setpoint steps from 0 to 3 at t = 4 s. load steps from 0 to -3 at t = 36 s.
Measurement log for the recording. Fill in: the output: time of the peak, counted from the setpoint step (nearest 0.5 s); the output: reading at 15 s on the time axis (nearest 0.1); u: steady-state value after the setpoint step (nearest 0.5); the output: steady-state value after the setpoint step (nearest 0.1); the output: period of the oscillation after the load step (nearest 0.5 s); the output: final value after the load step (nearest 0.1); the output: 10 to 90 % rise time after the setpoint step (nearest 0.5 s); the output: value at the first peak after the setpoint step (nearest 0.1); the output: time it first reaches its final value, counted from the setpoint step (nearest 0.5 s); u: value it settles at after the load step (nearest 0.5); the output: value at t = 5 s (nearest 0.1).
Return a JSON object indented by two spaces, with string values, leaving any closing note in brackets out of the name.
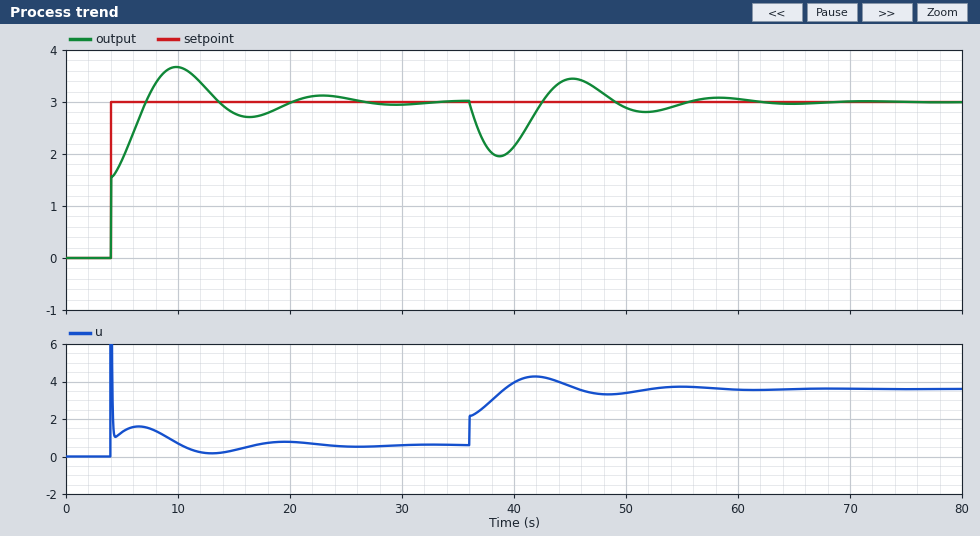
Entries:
{
  "the output: time of the peak, counted from the setpoint step": "6.0 s",
  "the output: reading at 15 s on the time axis": "2.8",
  "u: steady-state value after the setpoint step": "0.5",
  "the output: steady-state value after the setpoint step": "3.0",
  "the output: period of the oscillation after the load step": "13.0 s",
  "the output: final value after the load step": "3.0",
  "the output: 10 to 90 % rise time after the setpoint step": "2.5 s",
  "the output: value at the first peak after the setpoint step": "3.7",
  "the output: time it first reaches its final value, counted from the setpoint step": "3.0 s",
  "u: value it settles at after the load step": "3.5",
  "the output: value at t = 5 s": "1.9"
}
